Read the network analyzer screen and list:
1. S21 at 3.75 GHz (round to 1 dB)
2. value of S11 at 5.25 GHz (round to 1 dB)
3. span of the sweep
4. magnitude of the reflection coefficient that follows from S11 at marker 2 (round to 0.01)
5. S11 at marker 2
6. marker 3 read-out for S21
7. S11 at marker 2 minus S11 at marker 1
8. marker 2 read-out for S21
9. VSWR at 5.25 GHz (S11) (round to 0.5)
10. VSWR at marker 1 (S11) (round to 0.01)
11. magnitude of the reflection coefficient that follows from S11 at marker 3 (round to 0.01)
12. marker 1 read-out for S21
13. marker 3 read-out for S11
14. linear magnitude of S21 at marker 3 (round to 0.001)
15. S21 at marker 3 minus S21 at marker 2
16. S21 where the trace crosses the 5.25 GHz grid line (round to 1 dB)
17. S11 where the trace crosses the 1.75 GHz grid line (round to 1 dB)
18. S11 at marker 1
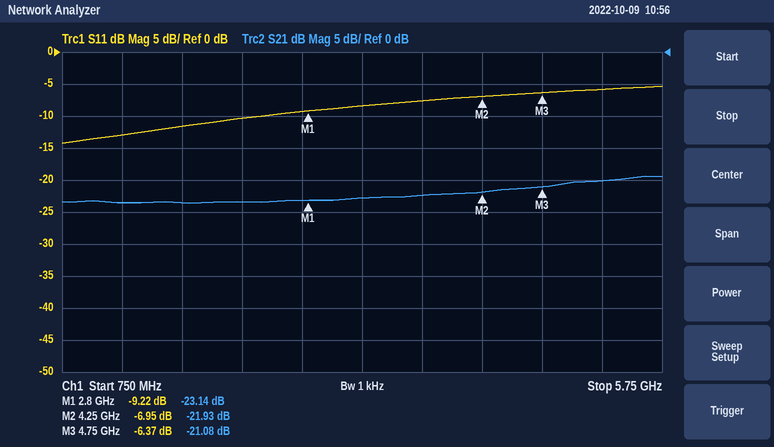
-22 dB
-6 dB
5 GHz
0.45
-6.95 dB
-21.08 dB
2.27 dB
-21.93 dB
3.0
2.06
0.48
-23.14 dB
-6.37 dB
0.088
0.85 dB
-20 dB
-12 dB
-9.22 dB
